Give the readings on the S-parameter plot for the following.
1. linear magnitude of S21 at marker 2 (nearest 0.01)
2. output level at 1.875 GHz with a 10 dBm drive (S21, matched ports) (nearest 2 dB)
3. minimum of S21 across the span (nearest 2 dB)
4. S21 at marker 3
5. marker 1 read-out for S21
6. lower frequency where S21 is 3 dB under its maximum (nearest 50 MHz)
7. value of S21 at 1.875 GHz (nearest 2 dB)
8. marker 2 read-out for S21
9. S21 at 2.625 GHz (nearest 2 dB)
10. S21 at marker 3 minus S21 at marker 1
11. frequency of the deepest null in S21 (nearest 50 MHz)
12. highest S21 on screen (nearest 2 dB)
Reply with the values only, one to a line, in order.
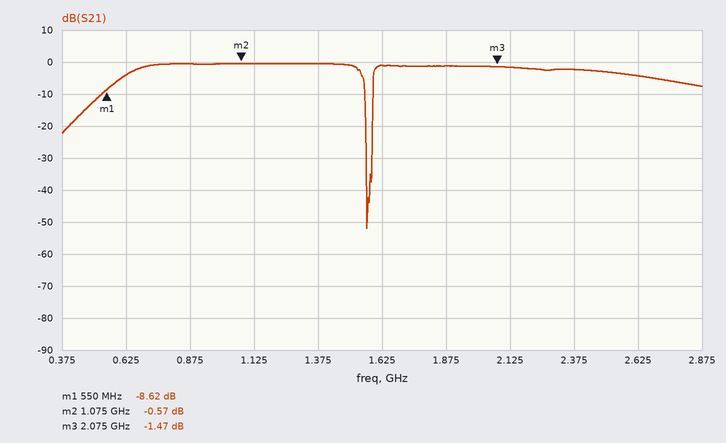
0.94
8 dBm
-52 dB
-1.47 dB
-8.62 dB
650 MHz
-2 dB
-0.57 dB
-4 dB
7.15 dB
1.55 GHz
0 dB
